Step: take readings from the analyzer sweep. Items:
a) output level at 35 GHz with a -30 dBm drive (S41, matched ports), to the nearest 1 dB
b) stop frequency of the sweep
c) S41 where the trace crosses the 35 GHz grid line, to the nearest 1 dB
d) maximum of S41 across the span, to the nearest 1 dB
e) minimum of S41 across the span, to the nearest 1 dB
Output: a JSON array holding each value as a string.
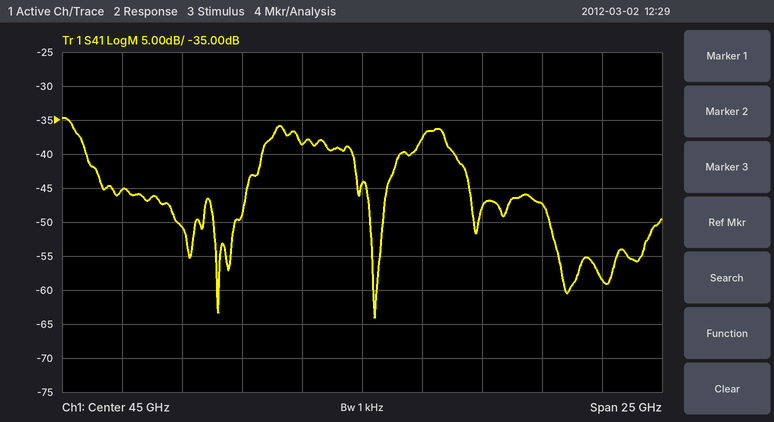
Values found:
["-75 dBm", "57.5 GHz", "-45 dB", "-35 dB", "-64 dB"]
